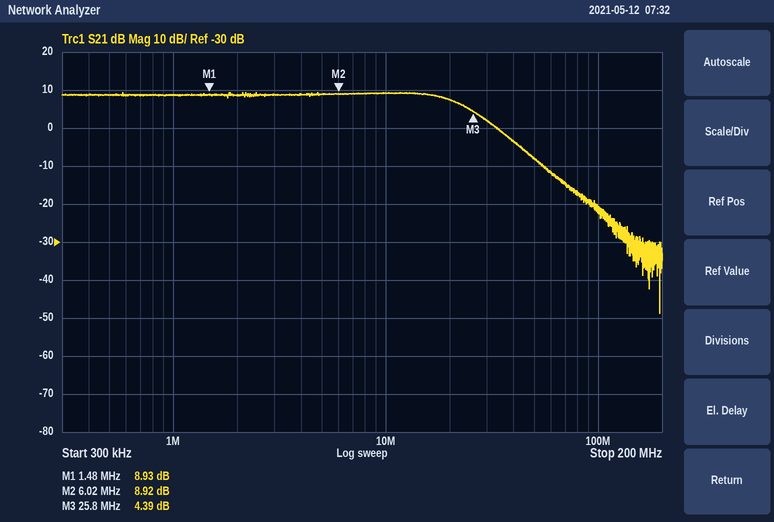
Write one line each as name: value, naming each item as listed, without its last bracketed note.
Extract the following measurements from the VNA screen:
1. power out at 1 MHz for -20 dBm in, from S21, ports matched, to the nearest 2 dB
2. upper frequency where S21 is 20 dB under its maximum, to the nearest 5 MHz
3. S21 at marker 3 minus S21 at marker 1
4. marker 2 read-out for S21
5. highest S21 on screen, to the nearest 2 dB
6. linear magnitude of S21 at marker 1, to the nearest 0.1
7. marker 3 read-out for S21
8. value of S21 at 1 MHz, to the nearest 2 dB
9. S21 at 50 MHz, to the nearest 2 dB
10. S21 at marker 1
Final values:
power out at 1 MHz for -20 dBm in, from S21, ports matched, to the nearest 2 dB: -12 dBm
upper frequency where S21 is 20 dB under its maximum, to the nearest 5 MHz: 55 MHz
S21 at marker 3 minus S21 at marker 1: -4.54 dB
marker 2 read-out for S21: 8.92 dB
highest S21 on screen, to the nearest 2 dB: 10 dB
linear magnitude of S21 at marker 1, to the nearest 0.1: 2.8
marker 3 read-out for S21: 4.39 dB
value of S21 at 1 MHz, to the nearest 2 dB: 8 dB
S21 at 50 MHz, to the nearest 2 dB: -8 dB
S21 at marker 1: 8.93 dB
